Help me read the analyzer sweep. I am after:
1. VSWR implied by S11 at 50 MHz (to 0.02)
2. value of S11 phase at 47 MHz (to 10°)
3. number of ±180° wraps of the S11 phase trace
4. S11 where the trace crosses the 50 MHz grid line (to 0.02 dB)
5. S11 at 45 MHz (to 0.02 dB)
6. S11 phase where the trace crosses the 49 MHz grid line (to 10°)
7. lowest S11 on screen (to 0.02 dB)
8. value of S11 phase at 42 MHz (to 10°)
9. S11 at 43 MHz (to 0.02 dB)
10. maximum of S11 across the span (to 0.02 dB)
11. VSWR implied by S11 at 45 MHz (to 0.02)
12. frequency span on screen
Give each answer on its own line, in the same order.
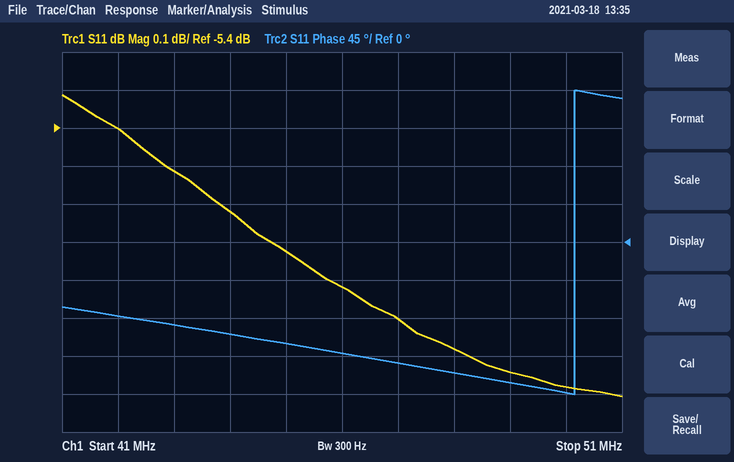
2.98
-140°
1
-6.08 dB
-5.72 dB
-170°
-6.10 dB
-90°
-5.52 dB
-5.32 dB
3.14
10 MHz
